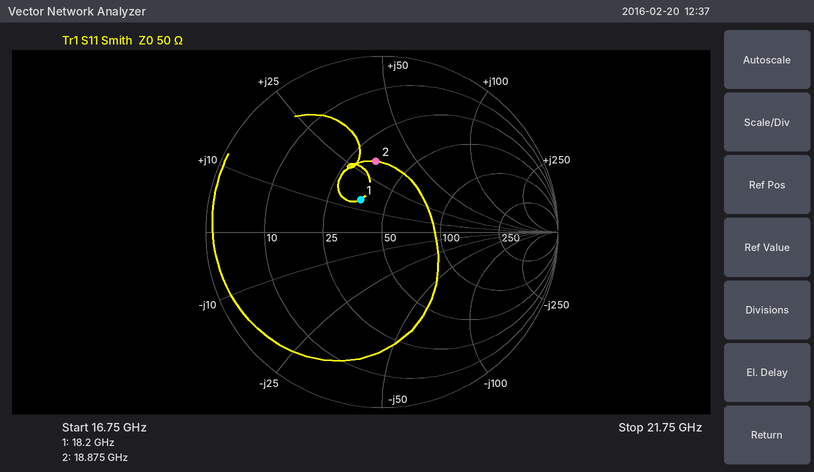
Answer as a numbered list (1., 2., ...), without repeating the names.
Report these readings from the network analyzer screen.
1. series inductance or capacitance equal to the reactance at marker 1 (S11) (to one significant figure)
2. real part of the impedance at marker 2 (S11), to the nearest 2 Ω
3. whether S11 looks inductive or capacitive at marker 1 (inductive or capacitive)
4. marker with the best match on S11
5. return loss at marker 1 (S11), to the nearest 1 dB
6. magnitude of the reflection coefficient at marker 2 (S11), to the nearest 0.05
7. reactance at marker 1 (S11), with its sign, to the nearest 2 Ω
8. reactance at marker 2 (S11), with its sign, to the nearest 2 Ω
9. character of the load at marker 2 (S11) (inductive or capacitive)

1. 100 pH
2. 34 Ω
3. inductive
4. marker 1
5. 13 dB
6. 0.40
7. +14 Ω
8. +32 Ω
9. inductive
